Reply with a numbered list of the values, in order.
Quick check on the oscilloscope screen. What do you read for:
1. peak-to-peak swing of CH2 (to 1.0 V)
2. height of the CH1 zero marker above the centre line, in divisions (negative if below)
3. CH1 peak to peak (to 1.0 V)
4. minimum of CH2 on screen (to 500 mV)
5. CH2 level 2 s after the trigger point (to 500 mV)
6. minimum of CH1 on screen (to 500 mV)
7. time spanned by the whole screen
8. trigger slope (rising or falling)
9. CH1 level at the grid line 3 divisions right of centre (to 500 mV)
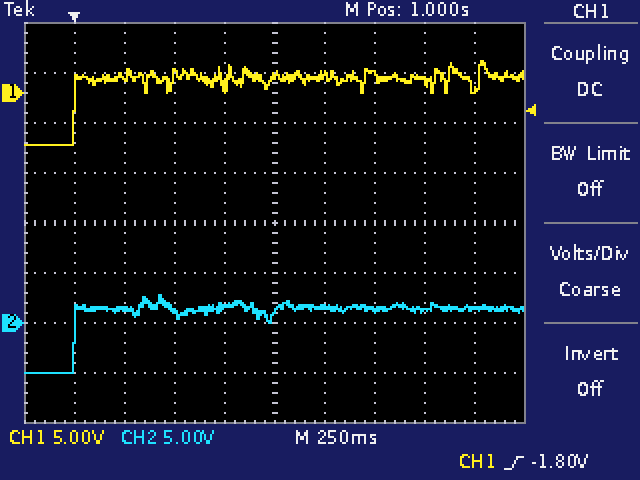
1. 8.0 V
2. +2.6 div
3. 8.0 V
4. -5.0 V
5. 1.5 V
6. -5.0 V
7. 2.5 s
8. rising
9. 1.0 V
